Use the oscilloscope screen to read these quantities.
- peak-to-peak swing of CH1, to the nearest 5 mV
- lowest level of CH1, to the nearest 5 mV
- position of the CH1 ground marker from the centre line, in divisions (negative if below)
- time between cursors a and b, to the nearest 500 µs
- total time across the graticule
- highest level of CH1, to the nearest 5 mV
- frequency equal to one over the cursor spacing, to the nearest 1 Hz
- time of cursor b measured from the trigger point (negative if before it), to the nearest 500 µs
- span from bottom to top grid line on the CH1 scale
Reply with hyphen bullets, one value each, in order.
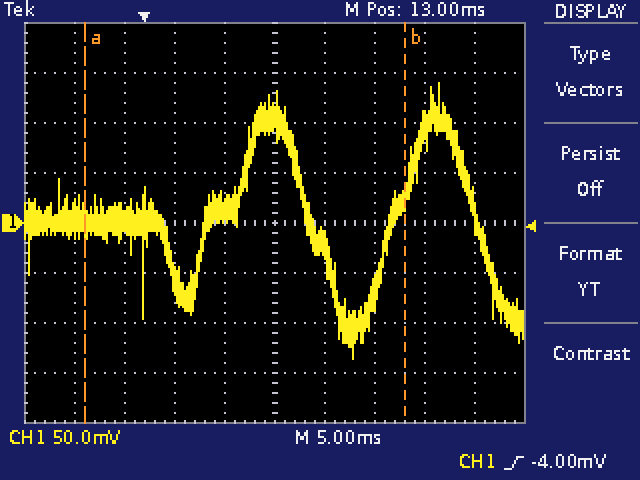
- 275 mV
- -135 mV
- 0.0 div
- 32.0 ms
- 50 ms
- 140 mV
- 31 Hz
- +26.0 ms
- 400 mV
